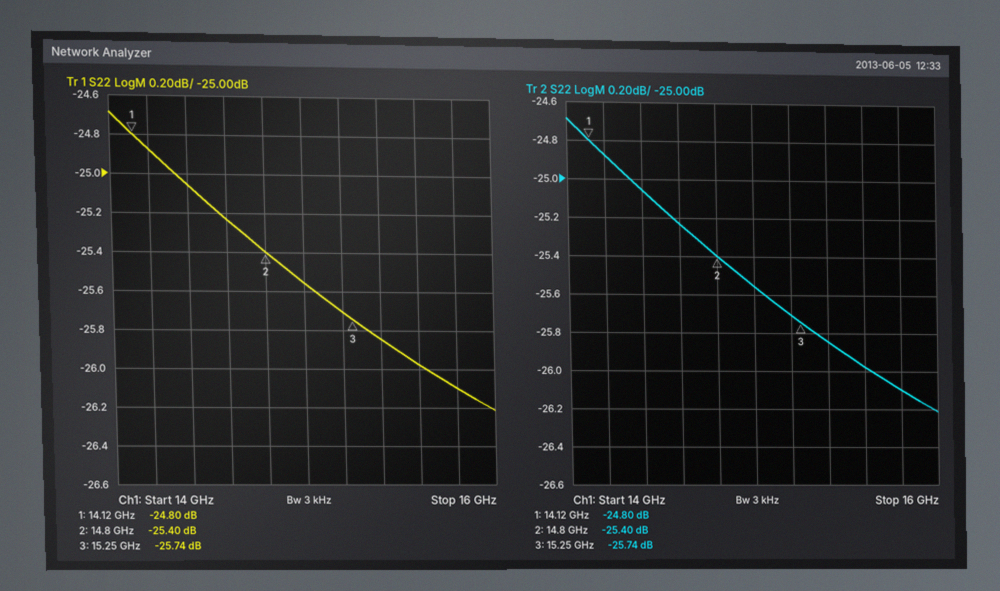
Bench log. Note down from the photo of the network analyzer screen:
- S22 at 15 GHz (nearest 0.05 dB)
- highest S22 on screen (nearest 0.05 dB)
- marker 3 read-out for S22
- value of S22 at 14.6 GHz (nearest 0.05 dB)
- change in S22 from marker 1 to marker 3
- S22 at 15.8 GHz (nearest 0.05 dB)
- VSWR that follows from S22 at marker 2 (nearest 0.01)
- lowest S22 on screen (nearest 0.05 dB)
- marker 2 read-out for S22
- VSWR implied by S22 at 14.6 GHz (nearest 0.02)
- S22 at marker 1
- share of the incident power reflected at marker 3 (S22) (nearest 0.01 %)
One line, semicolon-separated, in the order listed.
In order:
-25.55 dB; -24.70 dB; -25.74 dB; -25.25 dB; -0.94 dB; -26.10 dB; 1.11; -26.20 dB; -25.40 dB; 1.12; -24.80 dB; 0.27 %
